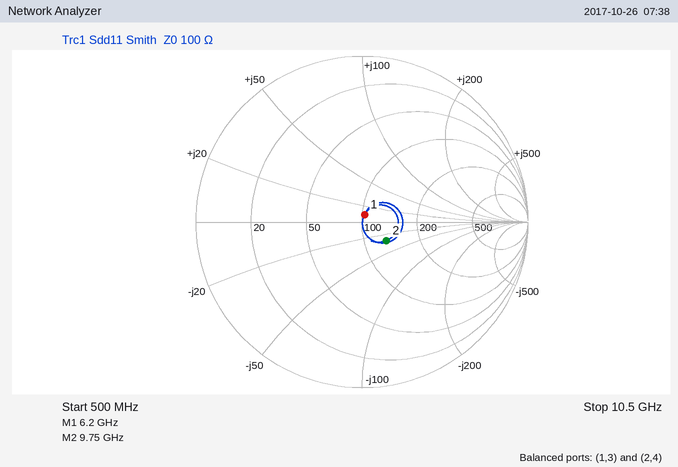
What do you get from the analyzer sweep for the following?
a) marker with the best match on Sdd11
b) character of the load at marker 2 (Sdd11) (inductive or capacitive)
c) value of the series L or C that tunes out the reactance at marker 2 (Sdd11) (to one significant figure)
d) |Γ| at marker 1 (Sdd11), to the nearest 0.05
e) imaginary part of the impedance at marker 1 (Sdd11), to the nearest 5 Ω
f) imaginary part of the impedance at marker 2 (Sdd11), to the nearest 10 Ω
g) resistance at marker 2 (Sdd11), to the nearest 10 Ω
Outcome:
marker 1
capacitive
500 pH
0.05
+10 Ω
-30 Ω
130 Ω
